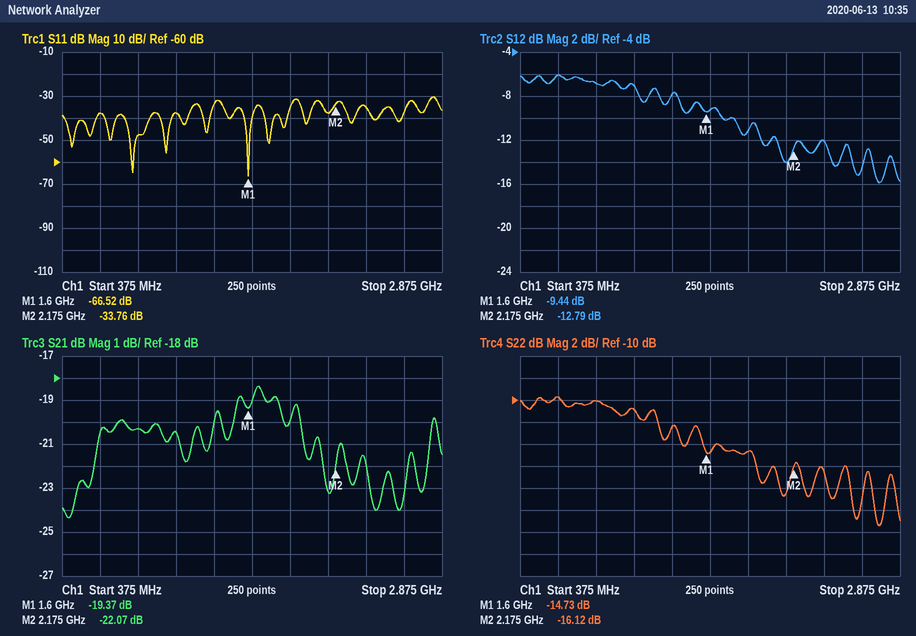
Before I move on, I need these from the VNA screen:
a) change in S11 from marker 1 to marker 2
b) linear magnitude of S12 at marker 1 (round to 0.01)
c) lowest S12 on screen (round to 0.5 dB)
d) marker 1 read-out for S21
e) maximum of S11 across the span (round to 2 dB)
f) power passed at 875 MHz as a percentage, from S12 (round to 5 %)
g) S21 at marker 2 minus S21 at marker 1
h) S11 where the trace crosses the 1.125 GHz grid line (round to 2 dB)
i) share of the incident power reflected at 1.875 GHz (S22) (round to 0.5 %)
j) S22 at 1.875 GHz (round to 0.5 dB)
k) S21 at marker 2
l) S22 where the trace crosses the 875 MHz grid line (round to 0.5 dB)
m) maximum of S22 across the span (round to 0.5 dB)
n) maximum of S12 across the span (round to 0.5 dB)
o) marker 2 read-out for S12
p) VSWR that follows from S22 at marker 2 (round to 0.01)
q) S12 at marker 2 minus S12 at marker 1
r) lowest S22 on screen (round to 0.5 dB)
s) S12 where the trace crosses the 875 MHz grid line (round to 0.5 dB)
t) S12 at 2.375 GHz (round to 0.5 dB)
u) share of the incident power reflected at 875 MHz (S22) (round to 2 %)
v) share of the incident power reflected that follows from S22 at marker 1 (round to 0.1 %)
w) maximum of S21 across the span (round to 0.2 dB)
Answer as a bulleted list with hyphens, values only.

- 32.76 dB
- 0.34
- -16.0 dB
- -19.37 dB
- -30 dB
- 20 %
- -2.70 dB
- -38 dB
- 3.5 %
- -14.5 dB
- -22.07 dB
- -10.0 dB
- -9.5 dB
- -6.0 dB
- -12.79 dB
- 1.37
- -3.35 dB
- -21.5 dB
- -7.0 dB
- -12.0 dB
- 10 %
- 3.4 %
- -18.4 dB
